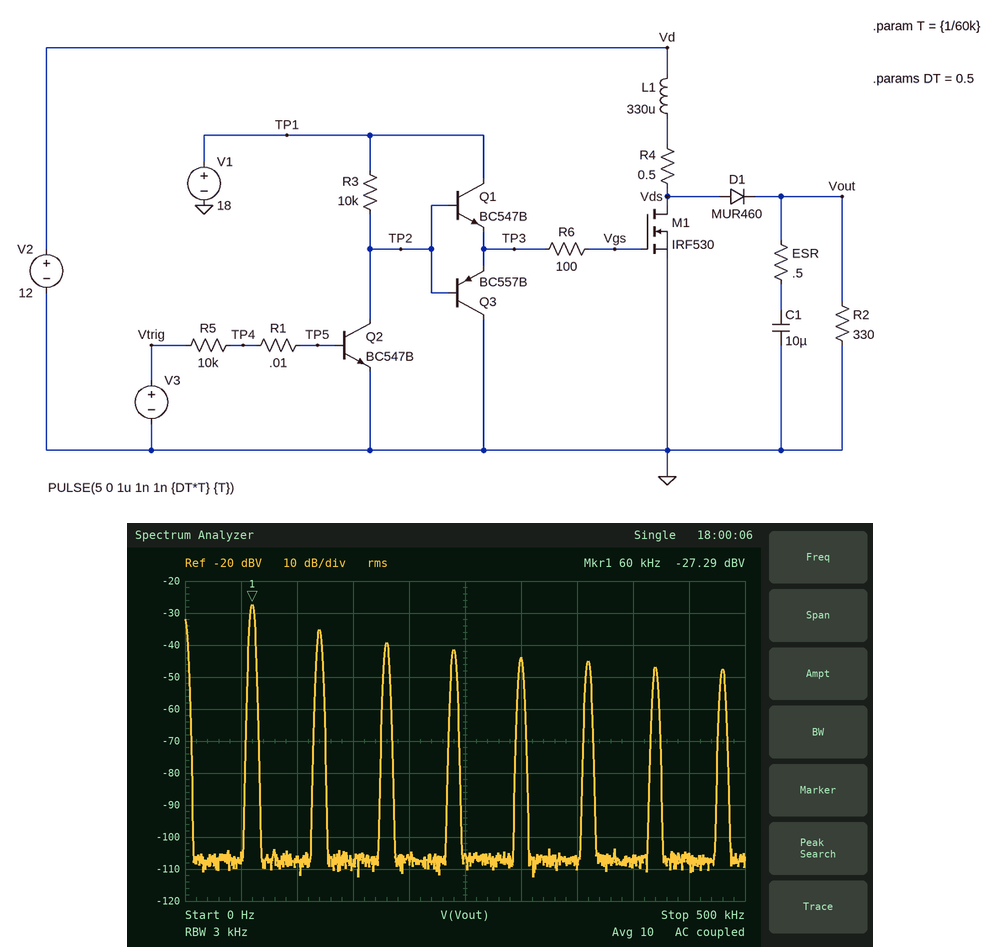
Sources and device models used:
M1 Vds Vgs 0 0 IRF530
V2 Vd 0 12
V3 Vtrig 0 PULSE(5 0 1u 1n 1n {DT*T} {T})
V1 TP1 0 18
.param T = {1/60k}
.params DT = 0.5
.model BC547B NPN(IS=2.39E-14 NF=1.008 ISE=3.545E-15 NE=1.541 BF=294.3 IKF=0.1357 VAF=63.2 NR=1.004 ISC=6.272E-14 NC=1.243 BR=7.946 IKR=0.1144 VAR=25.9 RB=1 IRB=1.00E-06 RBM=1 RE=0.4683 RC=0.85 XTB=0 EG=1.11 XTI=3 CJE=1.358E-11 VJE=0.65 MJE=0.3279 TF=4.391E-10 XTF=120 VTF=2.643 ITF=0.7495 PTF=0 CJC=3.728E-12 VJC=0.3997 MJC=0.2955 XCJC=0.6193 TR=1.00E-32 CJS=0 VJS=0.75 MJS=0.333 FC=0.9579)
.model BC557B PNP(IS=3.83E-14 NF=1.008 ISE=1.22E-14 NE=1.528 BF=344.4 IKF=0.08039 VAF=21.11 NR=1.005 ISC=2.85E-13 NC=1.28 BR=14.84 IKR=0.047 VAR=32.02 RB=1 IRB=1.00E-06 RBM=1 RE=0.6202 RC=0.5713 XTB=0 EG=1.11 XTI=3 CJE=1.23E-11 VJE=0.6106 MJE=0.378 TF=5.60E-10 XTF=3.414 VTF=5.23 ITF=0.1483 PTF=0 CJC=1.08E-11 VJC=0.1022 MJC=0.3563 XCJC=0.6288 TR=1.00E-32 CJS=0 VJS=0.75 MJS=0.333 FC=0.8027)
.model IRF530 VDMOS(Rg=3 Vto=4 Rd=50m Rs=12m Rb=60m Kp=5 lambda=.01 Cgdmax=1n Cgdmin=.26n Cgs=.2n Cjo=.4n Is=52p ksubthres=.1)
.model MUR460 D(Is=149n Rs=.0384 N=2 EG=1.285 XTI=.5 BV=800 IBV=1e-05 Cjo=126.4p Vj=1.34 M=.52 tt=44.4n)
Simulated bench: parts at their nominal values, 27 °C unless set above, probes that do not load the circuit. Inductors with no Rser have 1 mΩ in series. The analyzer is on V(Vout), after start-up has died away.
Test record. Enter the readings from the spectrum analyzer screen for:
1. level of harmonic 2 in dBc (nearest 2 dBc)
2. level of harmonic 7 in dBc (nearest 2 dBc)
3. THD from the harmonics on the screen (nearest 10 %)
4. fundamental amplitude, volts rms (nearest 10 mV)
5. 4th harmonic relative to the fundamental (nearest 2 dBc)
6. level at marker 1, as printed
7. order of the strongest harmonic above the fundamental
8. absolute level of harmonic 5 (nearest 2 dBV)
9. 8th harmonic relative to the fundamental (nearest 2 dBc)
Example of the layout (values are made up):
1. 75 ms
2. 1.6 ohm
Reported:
1. -8 dBc
2. -20 dBc
3. 60 %
4. 40 mV
5. -14 dBc
6. -27.29 dBV
7. 2
8. -44 dBV
9. -20 dBc
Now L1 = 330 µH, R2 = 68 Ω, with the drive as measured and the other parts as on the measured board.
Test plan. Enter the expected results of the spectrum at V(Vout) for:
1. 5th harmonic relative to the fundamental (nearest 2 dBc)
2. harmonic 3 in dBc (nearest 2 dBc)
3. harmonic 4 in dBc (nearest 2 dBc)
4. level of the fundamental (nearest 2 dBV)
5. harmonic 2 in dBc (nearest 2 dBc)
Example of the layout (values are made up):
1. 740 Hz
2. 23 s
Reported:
1. -16 dBc
2. -10 dBc
3. -24 dBc
4. -16 dBV
5. -20 dBc
